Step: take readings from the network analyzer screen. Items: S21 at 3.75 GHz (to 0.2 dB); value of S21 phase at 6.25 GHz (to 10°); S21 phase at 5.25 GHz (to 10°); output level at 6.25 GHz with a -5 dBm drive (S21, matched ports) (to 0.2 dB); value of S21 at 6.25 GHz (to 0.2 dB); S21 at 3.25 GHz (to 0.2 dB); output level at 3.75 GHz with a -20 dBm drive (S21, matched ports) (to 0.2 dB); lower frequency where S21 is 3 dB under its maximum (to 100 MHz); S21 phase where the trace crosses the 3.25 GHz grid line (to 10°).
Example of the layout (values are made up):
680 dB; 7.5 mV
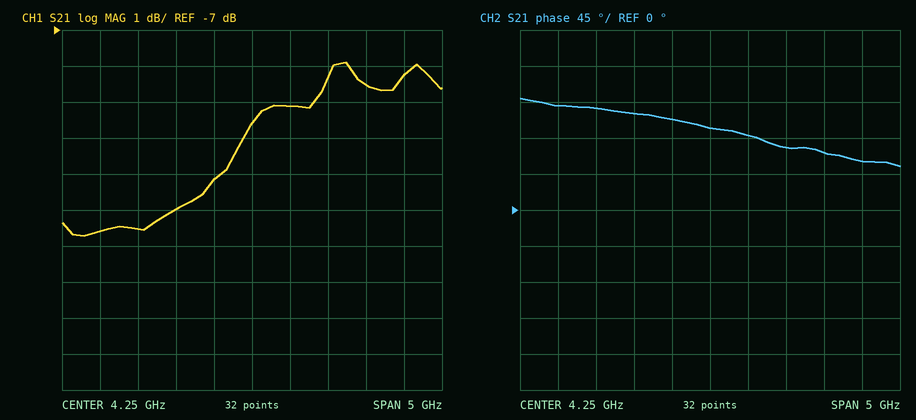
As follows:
-11.2 dB; 60°; 80°; -13.2 dBm; -8.2 dB; -12.0 dB; -31.2 dBm; 3.9 GHz; 120°
